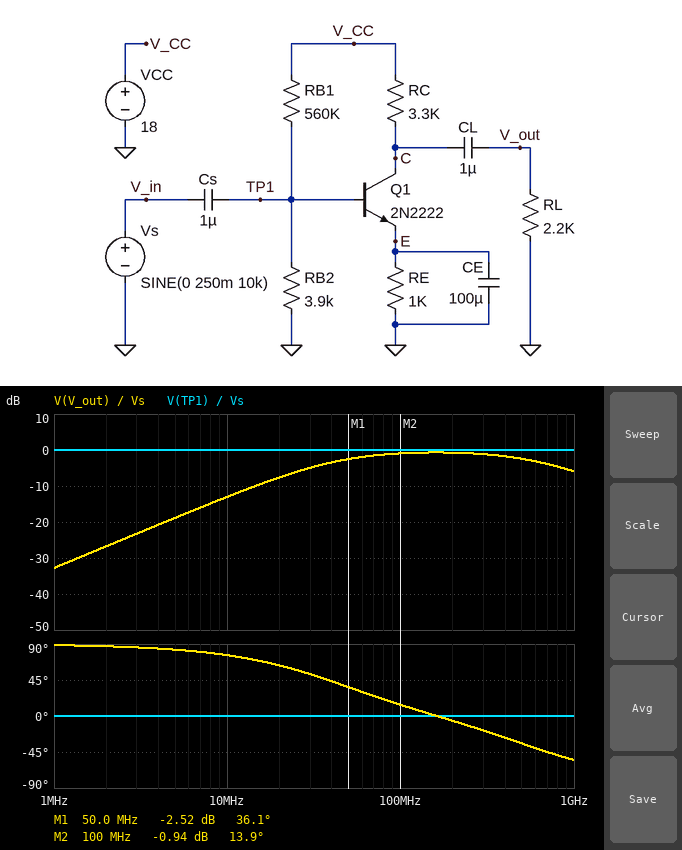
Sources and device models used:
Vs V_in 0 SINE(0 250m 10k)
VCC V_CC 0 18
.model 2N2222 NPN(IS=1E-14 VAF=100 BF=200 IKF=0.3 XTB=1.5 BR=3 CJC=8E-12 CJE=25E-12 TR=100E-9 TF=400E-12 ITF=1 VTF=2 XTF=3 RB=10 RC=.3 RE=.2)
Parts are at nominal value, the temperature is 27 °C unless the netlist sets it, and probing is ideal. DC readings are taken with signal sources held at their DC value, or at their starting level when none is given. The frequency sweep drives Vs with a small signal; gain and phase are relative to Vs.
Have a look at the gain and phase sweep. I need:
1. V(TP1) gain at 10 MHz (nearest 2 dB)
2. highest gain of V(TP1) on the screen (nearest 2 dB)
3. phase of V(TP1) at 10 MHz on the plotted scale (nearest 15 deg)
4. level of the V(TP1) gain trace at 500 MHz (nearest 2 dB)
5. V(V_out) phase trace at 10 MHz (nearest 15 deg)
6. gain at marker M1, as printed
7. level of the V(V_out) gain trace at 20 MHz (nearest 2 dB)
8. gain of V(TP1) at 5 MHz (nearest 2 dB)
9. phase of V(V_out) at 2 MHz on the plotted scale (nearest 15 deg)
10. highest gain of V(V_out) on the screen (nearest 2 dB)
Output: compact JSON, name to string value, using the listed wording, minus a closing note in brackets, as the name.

{"V(TP1) gain at 10 MHz": "0 dB", "highest gain of V(TP1) on the screen": "0 dB", "phase of V(TP1) at 10 MHz on the plotted scale": "0 deg", "level of the V(TP1) gain trace at 500 MHz": "0 dB", "V(V_out) phase trace at 10 MHz": "75 deg", "gain at marker M1, as printed": "-2.52 dB", "level of the V(V_out) gain trace at 20 MHz": "-8 dB", "gain of V(TP1) at 5 MHz": "0 dB", "phase of V(V_out) at 2 MHz on the plotted scale": "90 deg", "highest gain of V(V_out) on the screen": "0 dB"}
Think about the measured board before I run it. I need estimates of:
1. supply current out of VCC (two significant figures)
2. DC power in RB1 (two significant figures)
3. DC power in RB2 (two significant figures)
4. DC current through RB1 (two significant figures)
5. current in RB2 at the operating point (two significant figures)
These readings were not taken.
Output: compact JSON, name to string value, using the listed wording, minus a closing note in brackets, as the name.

{"supply current out of VCC": "32 µA", "DC power in RB1": "570 µW", "DC power in RB2": "4.0 µW", "DC current through RB1": "32 µA", "current in RB2 at the operating point": "32 µA"}
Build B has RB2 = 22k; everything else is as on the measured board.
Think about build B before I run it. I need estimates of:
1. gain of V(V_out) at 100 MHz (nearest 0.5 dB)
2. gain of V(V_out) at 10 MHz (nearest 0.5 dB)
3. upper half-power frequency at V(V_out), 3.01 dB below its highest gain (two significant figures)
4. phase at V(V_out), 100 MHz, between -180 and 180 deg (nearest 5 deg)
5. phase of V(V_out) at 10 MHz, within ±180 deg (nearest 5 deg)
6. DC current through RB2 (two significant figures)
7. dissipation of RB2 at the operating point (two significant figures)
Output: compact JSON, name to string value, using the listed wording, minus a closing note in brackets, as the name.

{"gain of V(V_out) at 100 MHz": "5.0 dB", "gain of V(V_out) at 10 MHz": "12.5 dB", "upper half-power frequency at V(V_out), 3.01 dB below its highest gain": "43 MHz", "phase at V(V_out), 100 MHz, between -180 and 180 deg": "70 deg", "phase of V(V_out) at 10 MHz, within ±180 deg": "160 deg", "DC current through RB2": "31 µA", "dissipation of RB2 at the operating point": "21 µW"}
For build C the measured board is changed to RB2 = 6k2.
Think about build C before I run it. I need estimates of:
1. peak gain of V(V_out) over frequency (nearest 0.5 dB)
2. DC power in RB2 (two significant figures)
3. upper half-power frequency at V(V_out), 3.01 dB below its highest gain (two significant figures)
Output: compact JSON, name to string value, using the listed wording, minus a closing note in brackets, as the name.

{"peak gain of V(V_out) over frequency": "-0.5 dB", "DC power in RB2": "6.3 µW", "upper half-power frequency at V(V_out), 3.01 dB below its highest gain": "650 MHz"}
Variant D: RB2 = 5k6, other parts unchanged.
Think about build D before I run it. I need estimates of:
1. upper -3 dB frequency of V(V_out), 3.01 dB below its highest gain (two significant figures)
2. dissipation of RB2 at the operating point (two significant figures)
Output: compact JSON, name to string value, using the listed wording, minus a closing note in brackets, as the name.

{"upper -3 dB frequency of V(V_out), 3.01 dB below its highest gain": "660 MHz", "dissipation of RB2 at the operating point": "5.7 µW"}
